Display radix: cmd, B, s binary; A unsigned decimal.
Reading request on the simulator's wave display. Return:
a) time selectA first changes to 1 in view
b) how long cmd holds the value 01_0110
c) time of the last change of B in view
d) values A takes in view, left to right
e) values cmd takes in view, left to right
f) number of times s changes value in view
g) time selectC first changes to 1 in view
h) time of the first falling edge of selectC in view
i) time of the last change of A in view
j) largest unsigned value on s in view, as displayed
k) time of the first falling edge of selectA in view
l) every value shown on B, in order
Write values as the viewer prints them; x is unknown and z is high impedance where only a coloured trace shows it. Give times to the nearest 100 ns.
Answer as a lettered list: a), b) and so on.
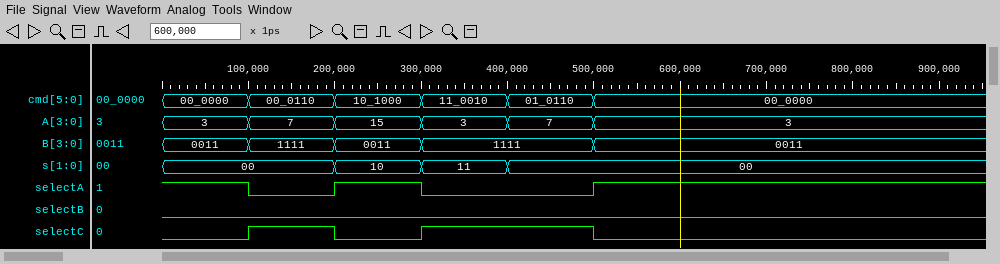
a) 200 ns
b) 100 ns
c) 500 ns
d) 3, 7, 15, 3, 7, 3
e) 00_0000, 00_0110, 10_1000, 11_0010, 01_0110, 00_0000
f) 3
g) 100 ns
h) 200 ns
i) 500 ns
j) 11
k) 100 ns
l) 0011, 1111, 0011, 1111, 0011
